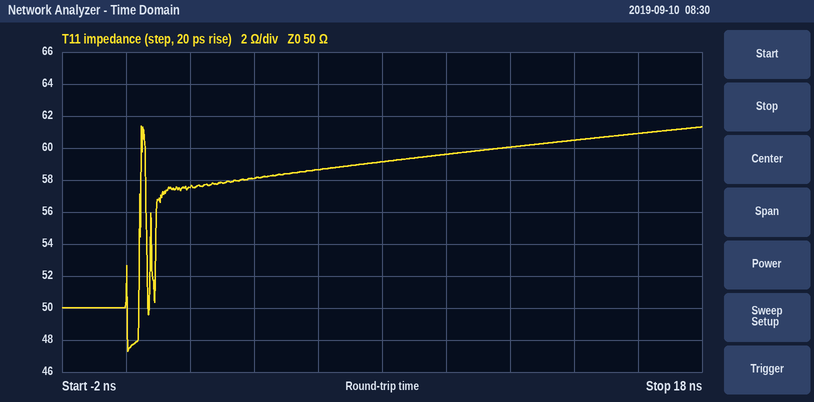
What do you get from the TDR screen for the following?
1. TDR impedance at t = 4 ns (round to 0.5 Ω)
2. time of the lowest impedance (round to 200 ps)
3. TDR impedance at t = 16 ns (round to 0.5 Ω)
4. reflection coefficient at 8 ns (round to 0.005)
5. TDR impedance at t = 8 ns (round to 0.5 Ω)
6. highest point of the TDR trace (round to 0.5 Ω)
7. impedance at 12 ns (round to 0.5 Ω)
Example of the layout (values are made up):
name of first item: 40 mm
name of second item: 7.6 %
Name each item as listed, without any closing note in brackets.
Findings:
TDR impedance at t = 4 ns: 58.0 Ω
time of the lowest impedance: 0.0 ns
TDR impedance at t = 16 ns: 61.0 Ω
reflection coefficient at 8 ns: +0.085
TDR impedance at t = 8 ns: 59.0 Ω
highest point of the TDR trace: 61.5 Ω
impedance at 12 ns: 60.0 Ω
